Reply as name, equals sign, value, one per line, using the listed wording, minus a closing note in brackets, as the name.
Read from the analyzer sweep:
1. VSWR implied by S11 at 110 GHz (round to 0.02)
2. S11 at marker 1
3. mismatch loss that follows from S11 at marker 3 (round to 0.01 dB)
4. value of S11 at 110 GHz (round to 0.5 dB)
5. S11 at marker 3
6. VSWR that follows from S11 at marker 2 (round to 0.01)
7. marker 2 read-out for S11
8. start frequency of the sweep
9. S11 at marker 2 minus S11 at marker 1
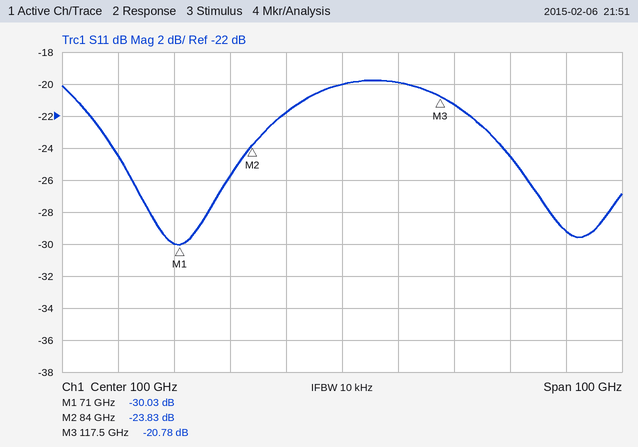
VSWR implied by S11 at 110 GHz = 1.22
S11 at marker 1 = -30.03 dB
mismatch loss that follows from S11 at marker 3 = 0.04 dB
value of S11 at 110 GHz = -20.0 dB
S11 at marker 3 = -20.78 dB
VSWR that follows from S11 at marker 2 = 1.14
marker 2 read-out for S11 = -23.83 dB
start frequency of the sweep = 50 GHz
S11 at marker 2 minus S11 at marker 1 = 6.20 dB
